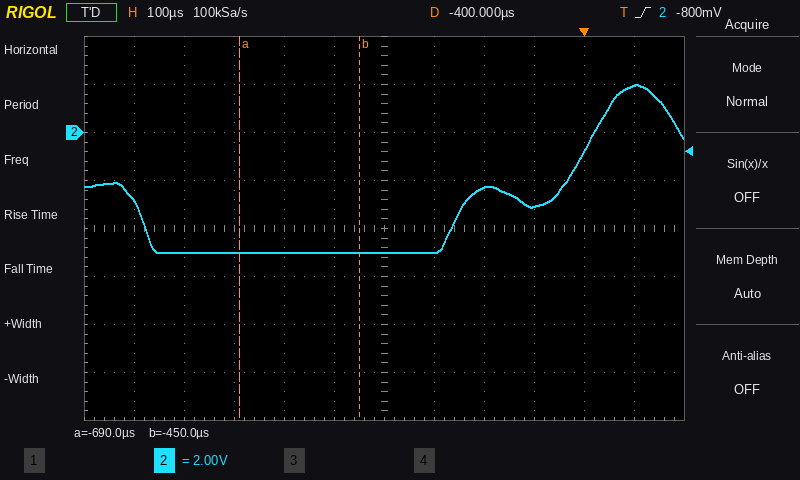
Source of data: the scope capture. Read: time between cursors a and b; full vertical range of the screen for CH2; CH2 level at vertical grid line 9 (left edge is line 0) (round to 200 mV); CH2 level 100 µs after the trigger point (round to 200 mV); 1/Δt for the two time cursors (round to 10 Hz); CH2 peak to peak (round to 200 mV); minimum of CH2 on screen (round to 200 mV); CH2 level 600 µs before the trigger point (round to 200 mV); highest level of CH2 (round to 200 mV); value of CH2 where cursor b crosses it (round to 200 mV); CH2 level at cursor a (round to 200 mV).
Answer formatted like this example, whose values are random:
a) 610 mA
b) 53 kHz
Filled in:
a) 240 µs
b) 16 V
c) -3.0 V
d) 2.0 V
e) 4.17 kHz
f) 7.0 V
g) -5.0 V
h) -5.0 V
i) 2.0 V
j) -5.0 V
k) -5.0 V
